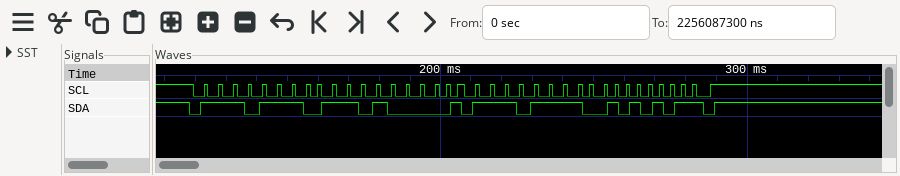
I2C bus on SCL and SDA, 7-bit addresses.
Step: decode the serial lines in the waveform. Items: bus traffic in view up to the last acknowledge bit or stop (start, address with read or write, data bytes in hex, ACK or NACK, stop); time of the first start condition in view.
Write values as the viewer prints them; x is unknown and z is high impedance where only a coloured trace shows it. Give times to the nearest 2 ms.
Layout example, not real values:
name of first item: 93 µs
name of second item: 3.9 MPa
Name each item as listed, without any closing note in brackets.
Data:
bus traffic in view up to the last acknowledge bit or stop: start, address 77 write ACK, D0 ACK, repeated start, address 77 read ACK, 55 NACK, stop
time of the first start condition in view: 118 ms
